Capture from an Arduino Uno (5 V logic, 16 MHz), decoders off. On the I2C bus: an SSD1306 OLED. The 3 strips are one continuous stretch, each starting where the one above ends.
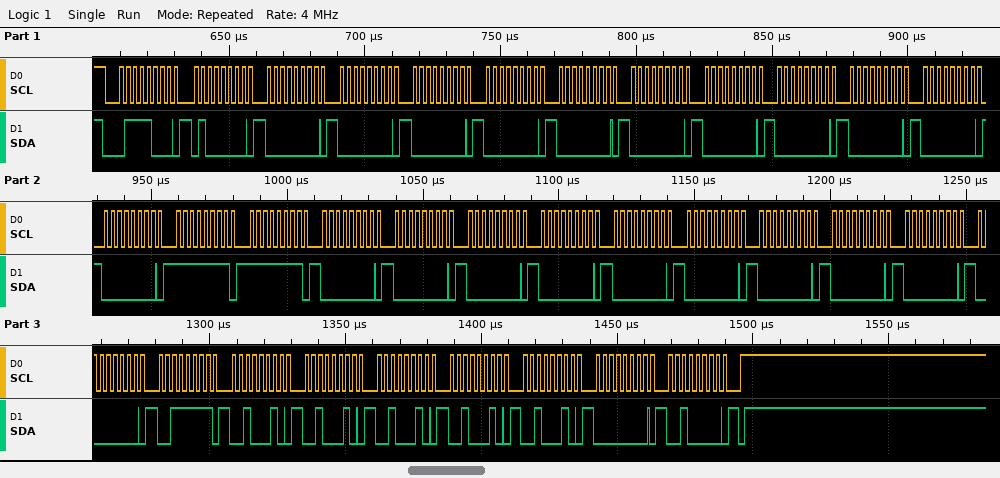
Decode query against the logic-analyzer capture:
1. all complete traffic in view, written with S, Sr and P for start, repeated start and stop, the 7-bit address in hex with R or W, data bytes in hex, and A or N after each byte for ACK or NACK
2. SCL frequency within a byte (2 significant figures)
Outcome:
S 3CW A 40 A 00 A 00 A 00 A 00 A 00 A 00 A 00 A 00 A 00 A 00 A 00 A FF A FF A 00 A 00 A 00 A 00 A 00 A 00 A 00 A 00 A 00 A 00 A 3F A 22 A 22 A 22 A 22 A 22 A 00 A 20 A P
400 kHz
